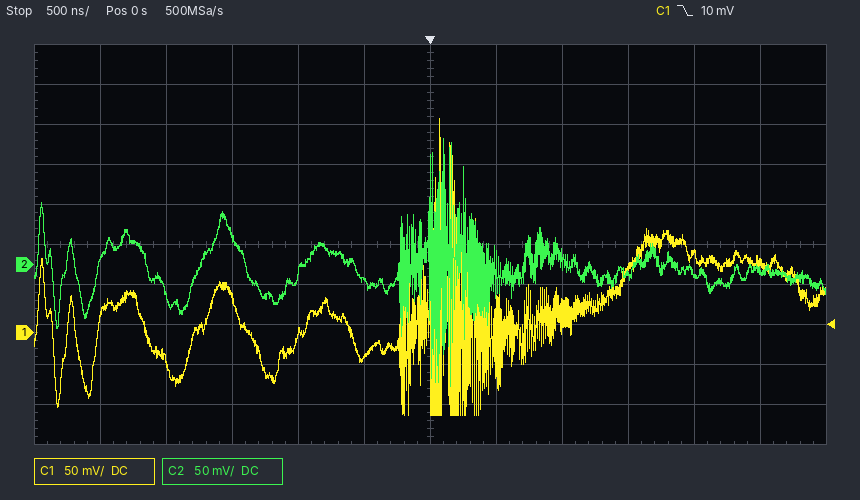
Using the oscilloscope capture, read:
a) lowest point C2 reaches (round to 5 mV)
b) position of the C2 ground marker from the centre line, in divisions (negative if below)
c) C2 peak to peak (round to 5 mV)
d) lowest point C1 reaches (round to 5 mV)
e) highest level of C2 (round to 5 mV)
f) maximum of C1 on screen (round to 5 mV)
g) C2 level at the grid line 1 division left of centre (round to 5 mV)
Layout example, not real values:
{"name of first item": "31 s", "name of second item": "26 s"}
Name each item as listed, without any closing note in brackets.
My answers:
{"lowest point C2 reaches": "-150 mV", "position of the C2 ground marker from the centre line, in divisions": "-0.5 div", "C2 peak to peak": "310 mV", "lowest point C1 reaches": "-105 mV", "highest level of C2": "160 mV", "maximum of C1 on screen": "270 mV", "C2 level at the grid line 1 division left of centre": "-20 mV"}
